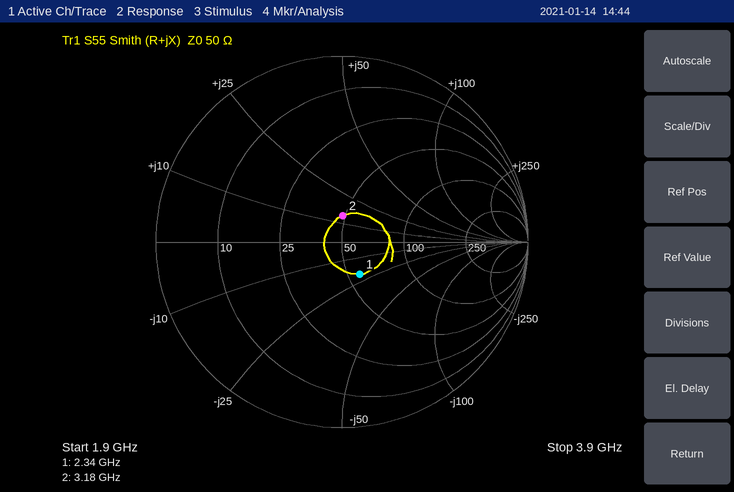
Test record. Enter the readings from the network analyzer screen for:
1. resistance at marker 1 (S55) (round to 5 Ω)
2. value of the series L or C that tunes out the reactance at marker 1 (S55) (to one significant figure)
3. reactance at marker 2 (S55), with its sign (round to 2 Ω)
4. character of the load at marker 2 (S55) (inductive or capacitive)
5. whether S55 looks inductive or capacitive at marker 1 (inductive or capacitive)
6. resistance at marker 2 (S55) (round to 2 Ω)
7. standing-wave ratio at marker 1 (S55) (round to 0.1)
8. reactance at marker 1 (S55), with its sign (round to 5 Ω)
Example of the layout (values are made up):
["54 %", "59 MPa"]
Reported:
["55 Ω", "1 nH", "+14 Ω", "inductive", "capacitive", "48 Ω", "1.5", "-20 Ω"]
